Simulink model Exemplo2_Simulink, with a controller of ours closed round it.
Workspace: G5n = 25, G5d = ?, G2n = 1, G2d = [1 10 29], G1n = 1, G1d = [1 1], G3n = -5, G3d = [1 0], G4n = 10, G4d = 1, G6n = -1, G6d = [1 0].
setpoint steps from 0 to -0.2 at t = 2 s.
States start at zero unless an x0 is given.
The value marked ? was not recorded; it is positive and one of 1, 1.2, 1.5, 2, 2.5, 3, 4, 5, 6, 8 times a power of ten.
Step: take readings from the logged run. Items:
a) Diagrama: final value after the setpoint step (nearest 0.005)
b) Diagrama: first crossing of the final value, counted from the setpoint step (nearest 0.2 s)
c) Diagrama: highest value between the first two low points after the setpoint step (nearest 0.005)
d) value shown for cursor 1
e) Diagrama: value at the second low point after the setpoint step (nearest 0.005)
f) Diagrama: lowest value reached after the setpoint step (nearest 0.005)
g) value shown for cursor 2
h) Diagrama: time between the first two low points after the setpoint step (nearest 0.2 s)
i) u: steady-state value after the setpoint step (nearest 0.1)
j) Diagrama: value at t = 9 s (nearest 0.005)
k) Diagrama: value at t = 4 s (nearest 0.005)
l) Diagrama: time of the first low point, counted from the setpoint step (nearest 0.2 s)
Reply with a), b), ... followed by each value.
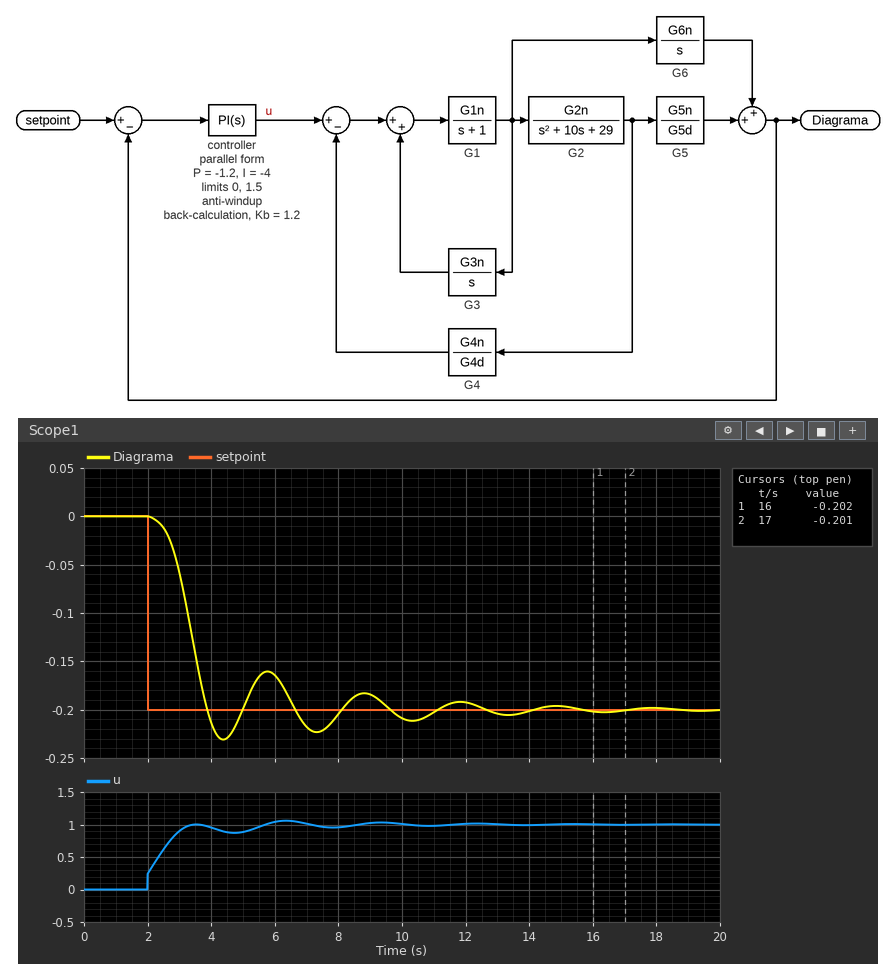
a) -0.200
b) 1.8 s
c) -0.160
d) -0.202
e) -0.225
f) -0.230
g) -0.201
h) 3.0 s
i) 1.0
j) -0.185
k) -0.215
l) 2.4 s
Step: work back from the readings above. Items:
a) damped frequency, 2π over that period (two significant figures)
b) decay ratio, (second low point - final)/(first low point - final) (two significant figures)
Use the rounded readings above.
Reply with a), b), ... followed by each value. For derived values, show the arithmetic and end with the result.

a) 2π / 3 = 2.1 rad/s
b) (-0.225 - (-0.2)) / (-0.23 - (-0.2)) = 0.83
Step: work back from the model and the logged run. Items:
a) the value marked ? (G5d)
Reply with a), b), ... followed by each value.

a) 2
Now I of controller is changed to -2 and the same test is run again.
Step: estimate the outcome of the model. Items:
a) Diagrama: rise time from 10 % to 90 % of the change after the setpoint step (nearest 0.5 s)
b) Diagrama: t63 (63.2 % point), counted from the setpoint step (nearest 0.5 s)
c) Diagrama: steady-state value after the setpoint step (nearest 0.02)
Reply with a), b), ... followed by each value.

a) 4.0 s
b) 2.0 s
c) -0.20
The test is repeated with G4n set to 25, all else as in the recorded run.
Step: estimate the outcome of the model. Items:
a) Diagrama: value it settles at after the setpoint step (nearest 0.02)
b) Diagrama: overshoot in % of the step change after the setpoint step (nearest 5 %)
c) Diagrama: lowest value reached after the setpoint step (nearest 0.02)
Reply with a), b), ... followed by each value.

a) -0.20
b) 10 %
c) -0.22
